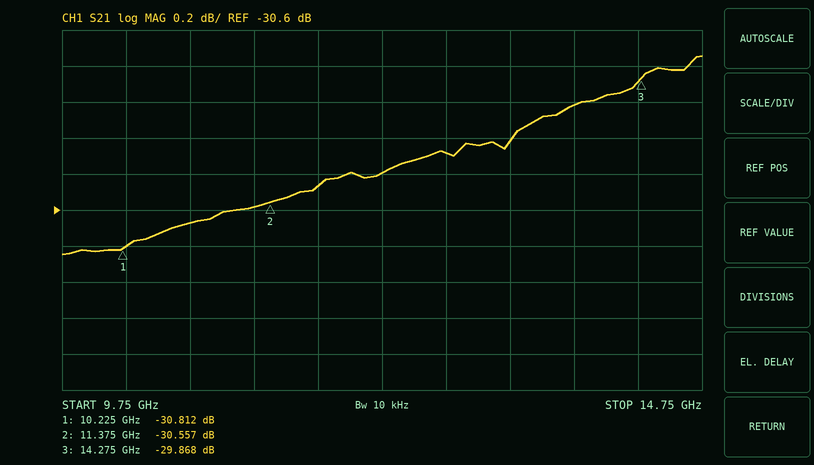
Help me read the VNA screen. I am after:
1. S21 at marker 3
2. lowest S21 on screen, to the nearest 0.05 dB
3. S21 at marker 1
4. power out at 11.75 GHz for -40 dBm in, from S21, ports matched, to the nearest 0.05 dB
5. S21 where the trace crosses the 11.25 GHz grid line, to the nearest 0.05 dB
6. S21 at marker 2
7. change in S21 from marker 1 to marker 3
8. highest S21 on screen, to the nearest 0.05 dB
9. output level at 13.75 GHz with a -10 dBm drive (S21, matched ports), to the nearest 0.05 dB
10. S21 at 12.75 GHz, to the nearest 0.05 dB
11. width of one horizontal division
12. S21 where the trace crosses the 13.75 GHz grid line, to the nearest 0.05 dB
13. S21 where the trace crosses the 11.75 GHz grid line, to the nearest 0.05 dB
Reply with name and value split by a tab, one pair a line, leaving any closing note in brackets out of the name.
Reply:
S21 at marker 3	-29.868 dB
lowest S21 on screen, to the nearest 0.05 dB	-30.85 dB
S21 at marker 1	-30.812 dB
power out at 11.75 GHz for -40 dBm in, from S21, ports matched, to the nearest 0.05 dB	-70.45 dBm
S21 where the trace crosses the 11.25 GHz grid line, to the nearest 0.05 dB	-30.60 dB
S21 at marker 2	-30.557 dB
change in S21 from marker 1 to marker 3	0.944 dB
highest S21 on screen, to the nearest 0.05 dB	-29.75 dB
output level at 13.75 GHz with a -10 dBm drive (S21, matched ports), to the nearest 0.05 dB	-40.00 dBm
S21 at 12.75 GHz, to the nearest 0.05 dB	-30.30 dB
width of one horizontal division	500 MHz
S21 where the trace crosses the 13.75 GHz grid line, to the nearest 0.05 dB	-30.00 dB
S21 where the trace crosses the 11.75 GHz grid line, to the nearest 0.05 dB	-30.45 dB
